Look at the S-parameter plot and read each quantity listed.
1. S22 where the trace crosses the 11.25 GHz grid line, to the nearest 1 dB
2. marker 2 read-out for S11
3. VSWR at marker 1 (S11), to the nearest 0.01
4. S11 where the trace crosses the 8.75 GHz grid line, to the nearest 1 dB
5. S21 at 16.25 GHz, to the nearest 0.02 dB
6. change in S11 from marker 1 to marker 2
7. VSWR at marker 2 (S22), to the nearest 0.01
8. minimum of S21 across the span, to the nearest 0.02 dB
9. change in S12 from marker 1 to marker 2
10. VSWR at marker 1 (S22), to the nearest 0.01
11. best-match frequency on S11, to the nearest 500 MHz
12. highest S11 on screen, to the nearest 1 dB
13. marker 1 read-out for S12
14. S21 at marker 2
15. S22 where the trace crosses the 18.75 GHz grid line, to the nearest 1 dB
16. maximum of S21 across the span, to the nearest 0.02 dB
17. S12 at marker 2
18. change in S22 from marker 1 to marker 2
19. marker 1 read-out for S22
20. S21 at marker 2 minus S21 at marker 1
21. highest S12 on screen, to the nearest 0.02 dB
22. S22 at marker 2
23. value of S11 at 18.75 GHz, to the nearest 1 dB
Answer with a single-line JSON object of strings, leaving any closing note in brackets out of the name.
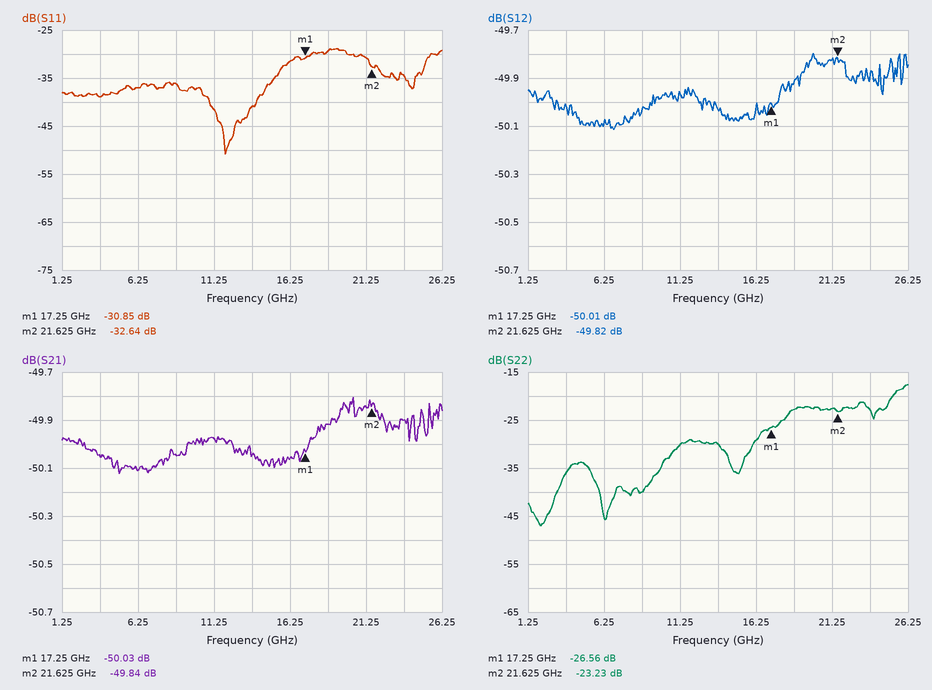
{"S22 where the trace crosses the 11.25 GHz grid line, to the nearest 1 dB": "-30 dB", "marker 2 read-out for S11": "-32.64 dB", "VSWR at marker 1 (S11), to the nearest 0.01": "1.06", "S11 where the trace crosses the 8.75 GHz grid line, to the nearest 1 dB": "-36 dB", "S21 at 16.25 GHz, to the nearest 0.02 dB": "-50.06 dB", "change in S11 from marker 1 to marker 2": "-1.79 dB", "VSWR at marker 2 (S22), to the nearest 0.01": "1.15", "minimum of S21 across the span, to the nearest 0.02 dB": "-50.12 dB", "change in S12 from marker 1 to marker 2": "0.19 dB", "VSWR at marker 1 (S22), to the nearest 0.01": "1.10", "best-match frequency on S11, to the nearest 500 MHz": "12.0 GHz", "highest S11 on screen, to the nearest 1 dB": "-29 dB", "marker 1 read-out for S12": "-50.01 dB", "S21 at marker 2": "-49.84 dB", "S22 where the trace crosses the 18.75 GHz grid line, to the nearest 1 dB": "-23 dB", "maximum of S21 across the span, to the nearest 0.02 dB": "-49.80 dB", "S12 at marker 2": "-49.82 dB", "change in S22 from marker 1 to marker 2": "3.33 dB", "marker 1 read-out for S22": "-26.56 dB", "S21 at marker 2 minus S21 at marker 1": "0.19 dB", "highest S12 on screen, to the nearest 0.02 dB": "-49.80 dB", "S22 at marker 2": "-23.23 dB", "value of S11 at 18.75 GHz, to the nearest 1 dB": "-29 dB"}
